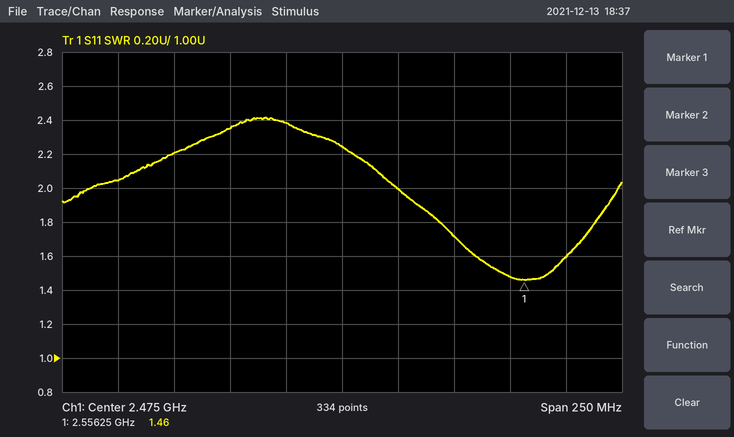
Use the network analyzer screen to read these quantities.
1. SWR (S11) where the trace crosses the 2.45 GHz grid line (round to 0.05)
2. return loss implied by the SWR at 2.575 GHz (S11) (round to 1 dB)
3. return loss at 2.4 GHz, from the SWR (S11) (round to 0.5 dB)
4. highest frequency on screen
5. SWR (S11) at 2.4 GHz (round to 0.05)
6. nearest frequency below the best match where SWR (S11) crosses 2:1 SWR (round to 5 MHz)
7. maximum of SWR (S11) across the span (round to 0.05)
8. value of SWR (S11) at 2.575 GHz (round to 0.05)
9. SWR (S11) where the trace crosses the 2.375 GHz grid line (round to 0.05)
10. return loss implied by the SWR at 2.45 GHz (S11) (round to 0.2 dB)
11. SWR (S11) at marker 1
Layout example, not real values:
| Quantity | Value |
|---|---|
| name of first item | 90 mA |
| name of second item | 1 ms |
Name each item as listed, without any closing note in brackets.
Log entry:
| Quantity | Value |
|---|---|
| SWR (S11) where the trace crosses the 2.45 GHz grid line | 2.40 |
| return loss implied by the SWR at 2.575 GHz (S11) | 13 dB |
| return loss at 2.4 GHz, from the SWR (S11) | 8.5 dB |
| highest frequency on screen | 2.6 GHz |
| SWR (S11) at 2.4 GHz | 2.20 |
| nearest frequency below the best match where SWR (S11) crosses 2:1 SWR | 2.500 GHz |
| maximum of SWR (S11) across the span | 2.40 |
| value of SWR (S11) at 2.575 GHz | 1.60 |
| SWR (S11) where the trace crosses the 2.375 GHz grid line | 2.05 |
| return loss implied by the SWR at 2.45 GHz (S11) | 7.8 dB |
| SWR (S11) at marker 1 | 1.46 |
